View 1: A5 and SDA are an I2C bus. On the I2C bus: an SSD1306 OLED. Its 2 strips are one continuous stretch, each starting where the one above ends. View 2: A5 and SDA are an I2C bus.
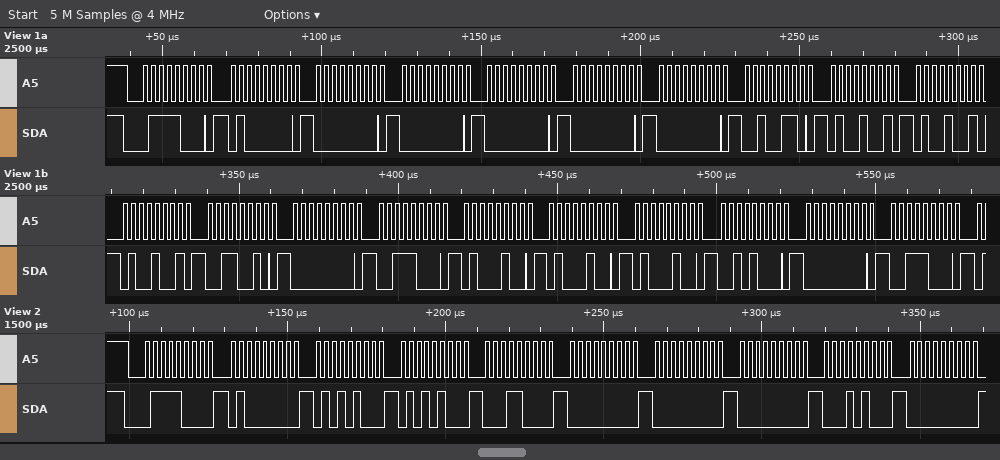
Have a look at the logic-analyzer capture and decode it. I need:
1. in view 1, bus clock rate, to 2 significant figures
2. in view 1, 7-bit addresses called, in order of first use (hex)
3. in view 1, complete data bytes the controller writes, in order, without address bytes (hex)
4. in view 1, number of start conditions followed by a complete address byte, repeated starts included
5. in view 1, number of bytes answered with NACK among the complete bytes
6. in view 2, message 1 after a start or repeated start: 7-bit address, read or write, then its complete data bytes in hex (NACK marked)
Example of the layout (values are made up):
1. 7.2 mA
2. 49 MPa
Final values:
1. 400 kHz
2. 0x3C
3. 40 00 00 00 00 00 26 49 49 49 32 00 38 44 44 44 28 00 38
4. 1
5. 0
6. 0x3C write: 40 54 54 18 00 00 00 14 00
